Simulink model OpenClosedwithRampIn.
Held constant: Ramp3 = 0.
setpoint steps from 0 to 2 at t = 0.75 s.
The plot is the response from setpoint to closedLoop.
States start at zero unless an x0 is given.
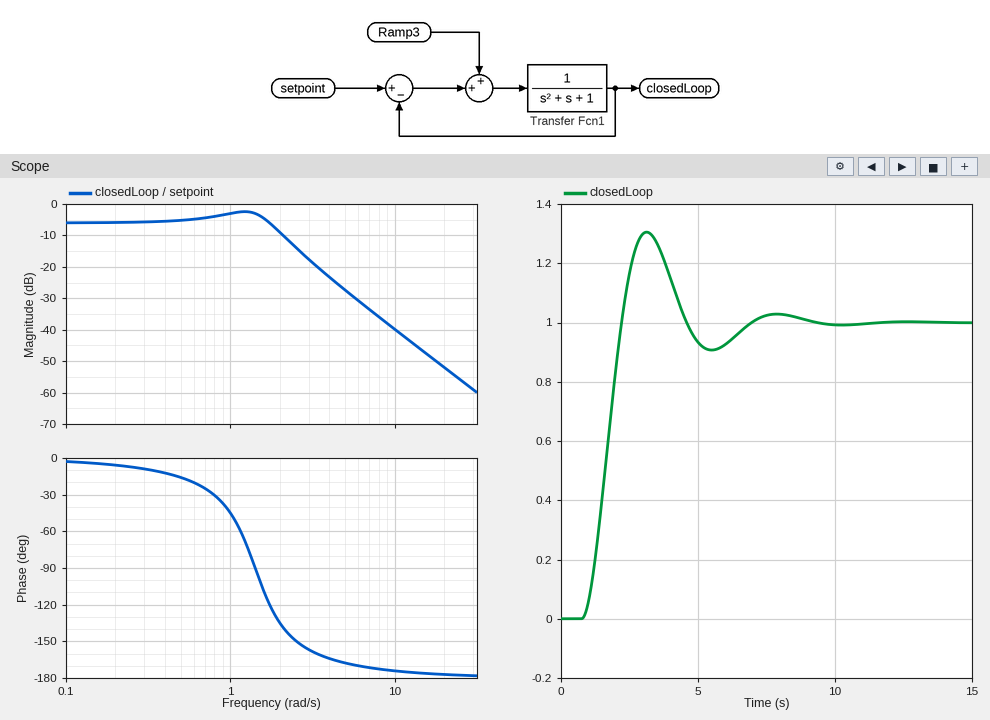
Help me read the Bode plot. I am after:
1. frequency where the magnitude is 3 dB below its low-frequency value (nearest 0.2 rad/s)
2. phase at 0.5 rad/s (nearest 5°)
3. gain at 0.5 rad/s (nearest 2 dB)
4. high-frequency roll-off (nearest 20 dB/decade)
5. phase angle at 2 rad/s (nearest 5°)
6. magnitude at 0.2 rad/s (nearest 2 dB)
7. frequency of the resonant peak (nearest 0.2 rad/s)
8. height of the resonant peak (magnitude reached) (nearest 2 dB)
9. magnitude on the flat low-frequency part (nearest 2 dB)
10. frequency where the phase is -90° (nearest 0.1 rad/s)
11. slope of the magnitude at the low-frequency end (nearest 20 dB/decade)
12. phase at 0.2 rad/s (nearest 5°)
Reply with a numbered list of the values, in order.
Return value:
1. 2.0 rad/s
2. -15°
3. -6 dB
4. -40 dB/decade
5. -135°
6. -6 dB
7. 1.2 rad/s
8. -2 dB
9. -6 dB
10. 1.4 rad/s
11. 0 dB/decade
12. -5°
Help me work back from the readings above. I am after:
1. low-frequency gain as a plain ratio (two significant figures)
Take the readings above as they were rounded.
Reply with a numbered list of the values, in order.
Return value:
1. 0.50
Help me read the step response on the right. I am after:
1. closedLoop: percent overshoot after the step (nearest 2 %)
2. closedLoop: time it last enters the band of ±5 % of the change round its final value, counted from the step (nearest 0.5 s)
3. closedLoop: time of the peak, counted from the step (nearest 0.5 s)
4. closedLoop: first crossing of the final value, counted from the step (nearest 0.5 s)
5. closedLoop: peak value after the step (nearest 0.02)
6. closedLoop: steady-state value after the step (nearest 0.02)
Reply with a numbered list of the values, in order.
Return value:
1. 30 %
2. 5.5 s
3. 2.5 s
4. 1.5 s
5. 1.30
6. 1.00
